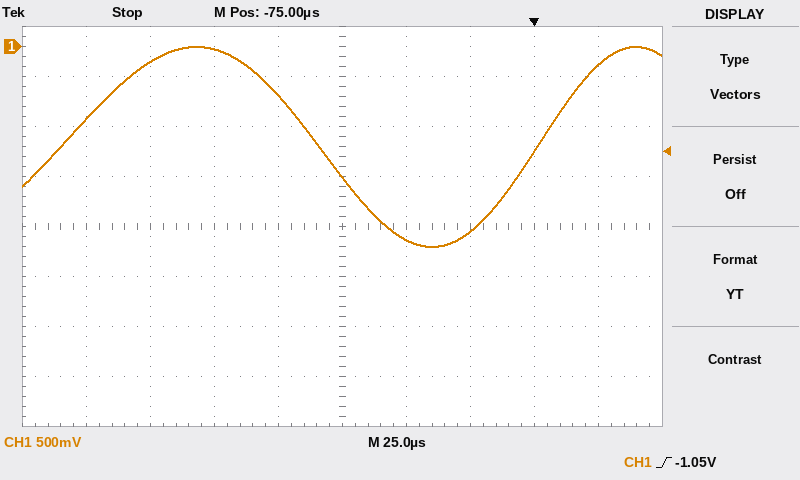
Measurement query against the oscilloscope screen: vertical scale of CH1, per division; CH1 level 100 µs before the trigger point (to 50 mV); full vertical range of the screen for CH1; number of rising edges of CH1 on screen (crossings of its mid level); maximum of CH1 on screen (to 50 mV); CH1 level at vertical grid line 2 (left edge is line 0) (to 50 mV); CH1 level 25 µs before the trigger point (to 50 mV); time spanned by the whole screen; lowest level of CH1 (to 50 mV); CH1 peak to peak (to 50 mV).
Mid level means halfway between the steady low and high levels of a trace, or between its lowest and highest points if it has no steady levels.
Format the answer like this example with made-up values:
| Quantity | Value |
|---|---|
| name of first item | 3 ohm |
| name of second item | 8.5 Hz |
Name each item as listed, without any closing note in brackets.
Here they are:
| Quantity | Value |
|---|---|
| vertical scale of CH1, per division | 500 mV |
| CH1 level 100 µs before the trigger point | -500 mV |
| full vertical range of the screen for CH1 | 4 V |
| number of rising edges of CH1 on screen | 2 |
| maximum of CH1 on screen | 0 mV |
| CH1 level at vertical grid line 2 (left edge is line 0) | -150 mV |
| CH1 level 25 µs before the trigger point | -1.85 V |
| time spanned by the whole screen | 250 µs |
| lowest level of CH1 | -2.00 V |
| CH1 peak to peak | 2.00 V |
